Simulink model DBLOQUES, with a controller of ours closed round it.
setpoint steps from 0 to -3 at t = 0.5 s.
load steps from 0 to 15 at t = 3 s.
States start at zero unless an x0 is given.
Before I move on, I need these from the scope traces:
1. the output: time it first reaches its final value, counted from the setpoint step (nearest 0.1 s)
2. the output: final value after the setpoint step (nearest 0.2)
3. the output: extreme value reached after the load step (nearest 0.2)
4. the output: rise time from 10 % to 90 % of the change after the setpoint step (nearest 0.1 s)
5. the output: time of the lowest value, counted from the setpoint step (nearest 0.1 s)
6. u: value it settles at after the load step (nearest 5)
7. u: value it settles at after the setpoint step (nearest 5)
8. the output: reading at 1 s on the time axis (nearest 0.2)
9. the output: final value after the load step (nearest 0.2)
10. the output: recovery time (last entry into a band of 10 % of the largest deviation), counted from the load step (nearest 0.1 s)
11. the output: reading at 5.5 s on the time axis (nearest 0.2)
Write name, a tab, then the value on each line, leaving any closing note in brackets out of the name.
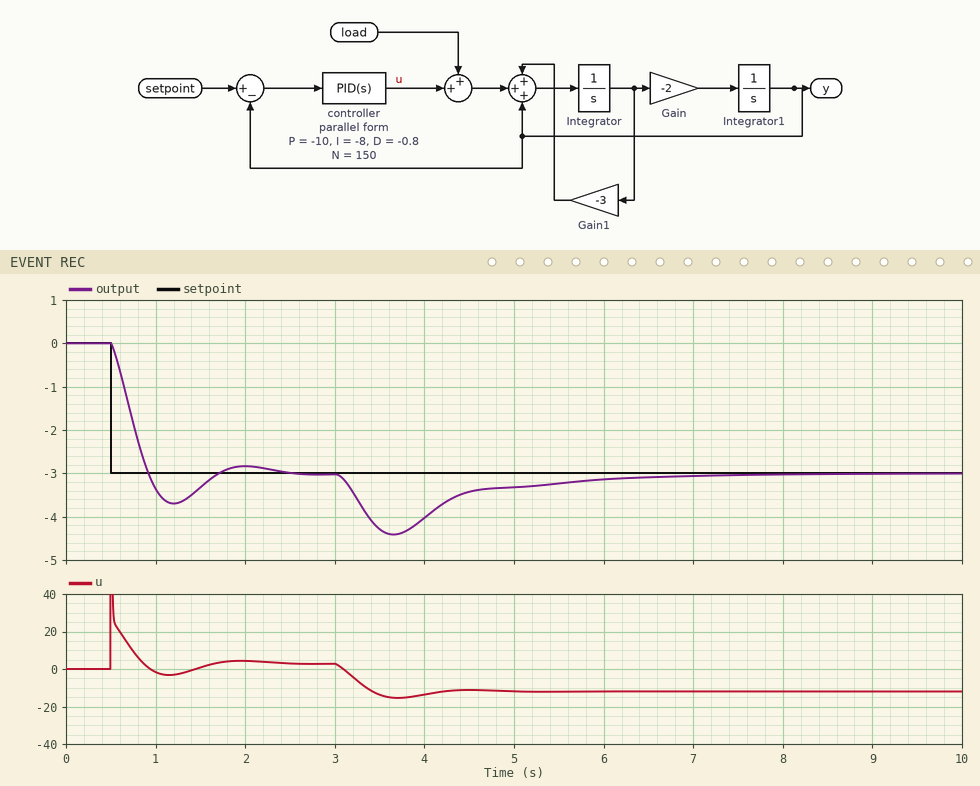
the output: time it first reaches its final value, counted from the setpoint step	0.4 s
the output: final value after the setpoint step	-3.0
the output: extreme value reached after the load step	-4.4
the output: rise time from 10 % to 90 % of the change after the setpoint step	0.3 s
the output: time of the lowest value, counted from the setpoint step	0.7 s
u: value it settles at after the load step	-10
u: value it settles at after the setpoint step	5
the output: reading at 1 s on the time axis	-3.4
the output: final value after the load step	-3.0
the output: recovery time (last entry into a band of 10 % of the largest deviation), counted from the load step	3.0 s
the output: reading at 5.5 s on the time axis	-3.2
